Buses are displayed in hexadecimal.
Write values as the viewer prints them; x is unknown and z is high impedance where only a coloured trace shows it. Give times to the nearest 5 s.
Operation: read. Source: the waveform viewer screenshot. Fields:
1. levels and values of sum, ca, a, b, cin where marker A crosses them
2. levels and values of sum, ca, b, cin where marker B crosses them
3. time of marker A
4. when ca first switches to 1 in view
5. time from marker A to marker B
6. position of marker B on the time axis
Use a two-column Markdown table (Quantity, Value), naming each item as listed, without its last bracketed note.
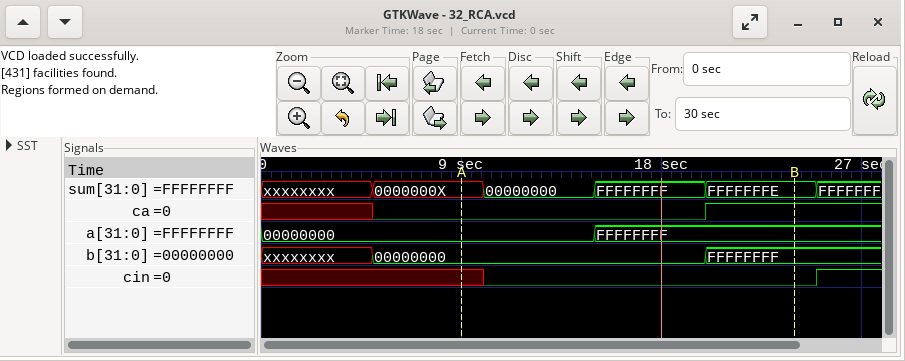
| Quantity | Value |
|---|---|
| levels and values of sum, ca, a, b, cin where marker A crosses them | sum=0000000X, ca=0, a=00000000, b=00000000, cin=x |
| levels and values of sum, ca, b, cin where marker B crosses them | sum=FFFFFFFE, ca=1, b=FFFFFFFF, cin=0 |
| time of marker A | 10 s |
| when ca first switches to 1 in view | 20 s |
| time from marker A to marker B | 15 s |
| position of marker B on the time axis | 25 s |
